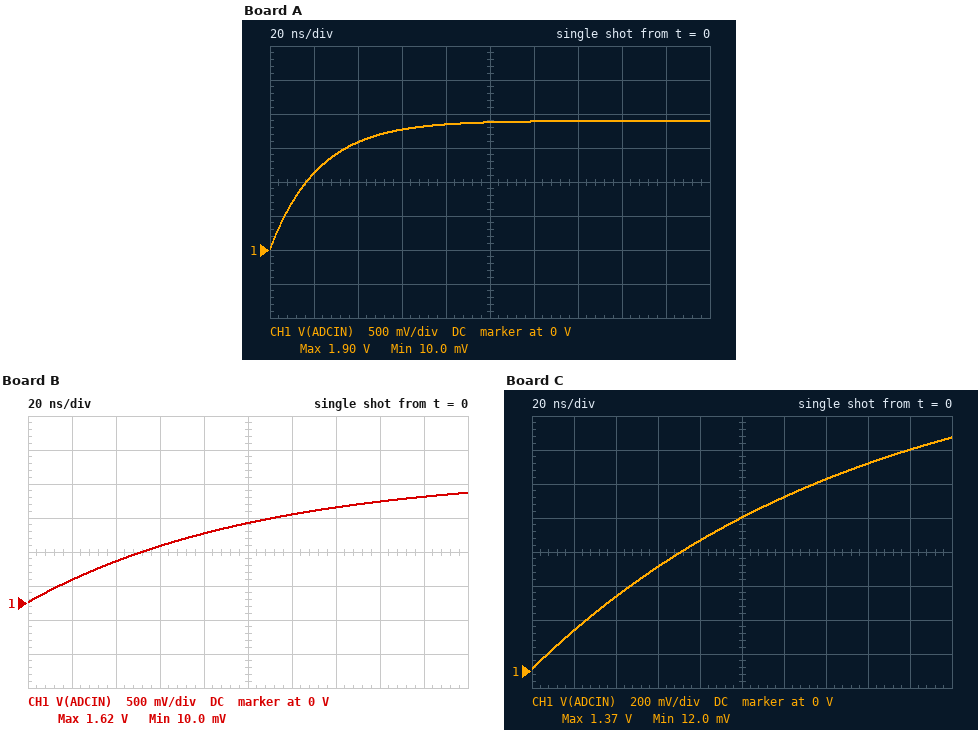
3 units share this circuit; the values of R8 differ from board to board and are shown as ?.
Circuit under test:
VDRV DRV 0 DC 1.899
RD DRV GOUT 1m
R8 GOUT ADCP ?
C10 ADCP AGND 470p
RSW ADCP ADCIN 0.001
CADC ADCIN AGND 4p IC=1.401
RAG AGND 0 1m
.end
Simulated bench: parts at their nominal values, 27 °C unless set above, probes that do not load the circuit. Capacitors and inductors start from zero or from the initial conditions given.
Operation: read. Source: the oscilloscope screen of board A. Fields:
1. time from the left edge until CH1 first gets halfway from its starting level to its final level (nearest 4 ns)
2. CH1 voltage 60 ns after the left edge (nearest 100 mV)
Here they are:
16 ns
1.8 V
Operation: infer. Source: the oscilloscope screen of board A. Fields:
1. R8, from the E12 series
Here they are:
47 Ω
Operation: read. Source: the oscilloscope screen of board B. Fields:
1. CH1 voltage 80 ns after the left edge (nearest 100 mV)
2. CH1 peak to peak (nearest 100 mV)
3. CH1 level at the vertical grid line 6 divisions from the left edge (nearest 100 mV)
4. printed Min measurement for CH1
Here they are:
1.0 V
1.6 V
1.3 V
10.0 mV
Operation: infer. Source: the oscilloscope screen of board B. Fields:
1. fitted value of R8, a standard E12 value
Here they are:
220 Ω
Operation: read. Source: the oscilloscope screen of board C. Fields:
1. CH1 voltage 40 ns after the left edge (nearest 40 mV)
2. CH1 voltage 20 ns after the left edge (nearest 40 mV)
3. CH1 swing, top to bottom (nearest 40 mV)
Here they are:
440 mV
240 mV
1.36 V
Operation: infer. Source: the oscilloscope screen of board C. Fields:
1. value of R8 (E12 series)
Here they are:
330 Ω
